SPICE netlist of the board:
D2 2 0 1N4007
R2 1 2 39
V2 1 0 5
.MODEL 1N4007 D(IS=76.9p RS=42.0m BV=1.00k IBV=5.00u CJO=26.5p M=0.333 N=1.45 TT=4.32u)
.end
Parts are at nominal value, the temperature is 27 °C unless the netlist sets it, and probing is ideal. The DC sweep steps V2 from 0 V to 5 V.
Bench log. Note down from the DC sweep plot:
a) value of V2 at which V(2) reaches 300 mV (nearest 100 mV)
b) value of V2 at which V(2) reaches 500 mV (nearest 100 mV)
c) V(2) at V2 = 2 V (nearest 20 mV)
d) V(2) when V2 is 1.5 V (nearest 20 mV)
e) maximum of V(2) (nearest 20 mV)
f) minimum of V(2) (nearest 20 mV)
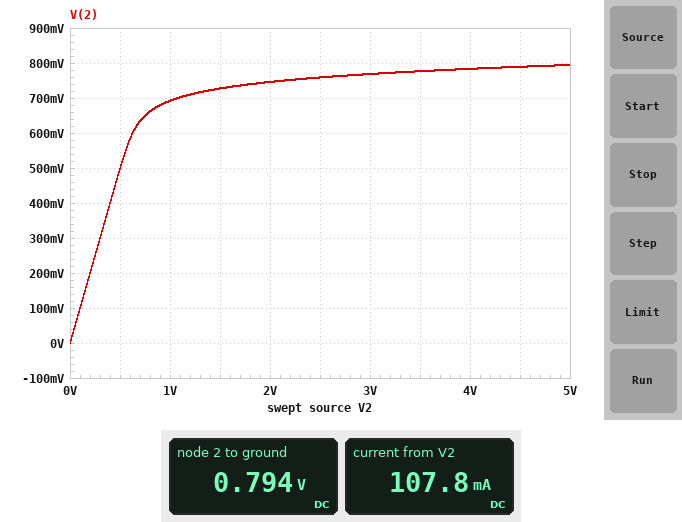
300 mV
500 mV
740 mV
720 mV
800 mV
0 V
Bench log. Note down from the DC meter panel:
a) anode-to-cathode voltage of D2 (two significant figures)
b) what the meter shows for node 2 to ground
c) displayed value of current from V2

790 mV
0.794 V
107.8 mA
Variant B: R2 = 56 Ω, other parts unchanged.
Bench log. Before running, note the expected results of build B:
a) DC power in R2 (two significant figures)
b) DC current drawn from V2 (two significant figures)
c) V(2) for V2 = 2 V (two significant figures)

320 mW
75 mA
730 mV
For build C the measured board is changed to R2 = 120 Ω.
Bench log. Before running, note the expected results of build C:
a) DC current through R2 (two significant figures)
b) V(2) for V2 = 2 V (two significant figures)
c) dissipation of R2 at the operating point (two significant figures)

35 mA
700 mV
150 mW
